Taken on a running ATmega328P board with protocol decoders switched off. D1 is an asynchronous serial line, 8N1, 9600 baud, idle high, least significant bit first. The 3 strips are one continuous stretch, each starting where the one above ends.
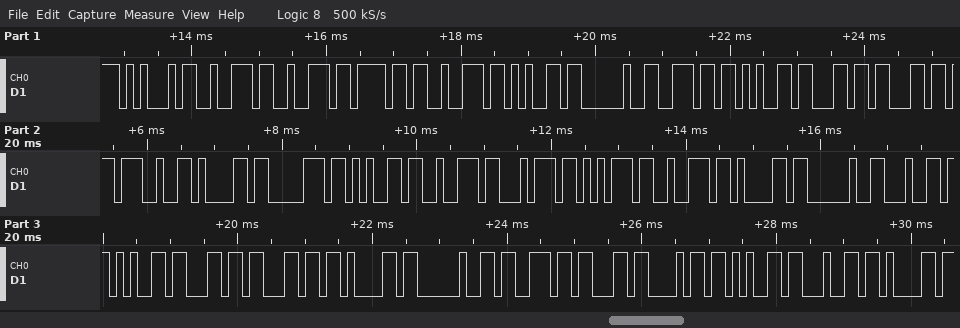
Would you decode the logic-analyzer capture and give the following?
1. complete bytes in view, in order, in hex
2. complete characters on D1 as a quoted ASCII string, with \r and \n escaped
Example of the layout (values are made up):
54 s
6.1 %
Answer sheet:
45 72 72 6F 72 65 20 6E 65 6C 6C 27 61 70 65 72 74 75 72 61 20 64 65 6C 6C 61 20 73 63 68 65 64 61
"Errore nell'apertura della scheda"
